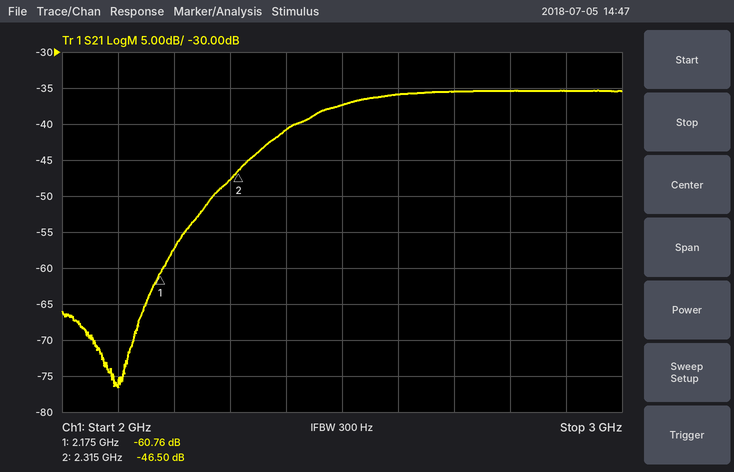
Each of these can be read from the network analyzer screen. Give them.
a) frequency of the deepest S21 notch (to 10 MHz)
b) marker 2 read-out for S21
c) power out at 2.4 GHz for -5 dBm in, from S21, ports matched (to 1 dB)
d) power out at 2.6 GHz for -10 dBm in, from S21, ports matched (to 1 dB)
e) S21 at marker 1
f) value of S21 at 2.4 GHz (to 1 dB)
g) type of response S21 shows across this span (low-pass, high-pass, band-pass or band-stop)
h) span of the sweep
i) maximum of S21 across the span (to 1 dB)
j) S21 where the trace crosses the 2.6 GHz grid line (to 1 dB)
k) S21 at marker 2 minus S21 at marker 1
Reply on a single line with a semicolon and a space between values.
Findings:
2.10 GHz; -46.50 dB; -46 dBm; -46 dBm; -60.76 dB; -41 dB; high-pass; 1 GHz; -35 dB; -36 dB; 14.26 dB
